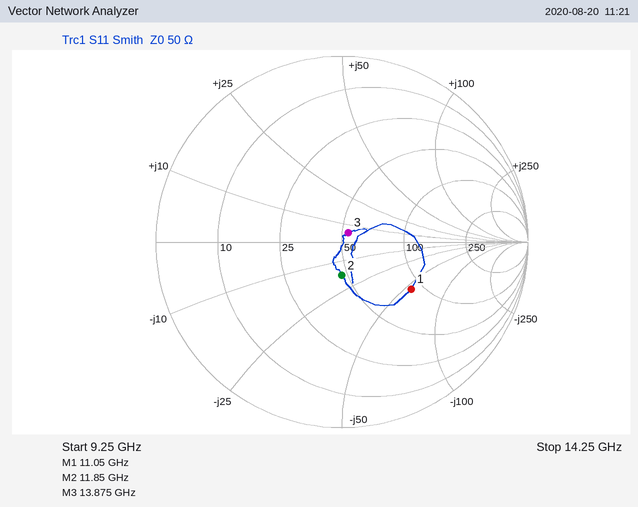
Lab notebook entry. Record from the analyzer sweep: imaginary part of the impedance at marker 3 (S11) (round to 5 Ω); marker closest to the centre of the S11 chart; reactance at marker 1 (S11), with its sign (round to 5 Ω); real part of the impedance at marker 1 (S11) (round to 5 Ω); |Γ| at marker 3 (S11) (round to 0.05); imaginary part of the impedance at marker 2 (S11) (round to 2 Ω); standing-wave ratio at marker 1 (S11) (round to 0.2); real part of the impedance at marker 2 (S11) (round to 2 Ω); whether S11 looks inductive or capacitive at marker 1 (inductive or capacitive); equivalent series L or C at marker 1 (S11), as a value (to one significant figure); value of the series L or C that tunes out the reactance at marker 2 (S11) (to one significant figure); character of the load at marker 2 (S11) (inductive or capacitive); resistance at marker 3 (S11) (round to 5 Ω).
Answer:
+5 Ω
marker 3
-55 Ω
85 Ω
0.05
-18 Ω
2.6
46 Ω
capacitive
300 fF
200 pH
capacitive
55 Ω
